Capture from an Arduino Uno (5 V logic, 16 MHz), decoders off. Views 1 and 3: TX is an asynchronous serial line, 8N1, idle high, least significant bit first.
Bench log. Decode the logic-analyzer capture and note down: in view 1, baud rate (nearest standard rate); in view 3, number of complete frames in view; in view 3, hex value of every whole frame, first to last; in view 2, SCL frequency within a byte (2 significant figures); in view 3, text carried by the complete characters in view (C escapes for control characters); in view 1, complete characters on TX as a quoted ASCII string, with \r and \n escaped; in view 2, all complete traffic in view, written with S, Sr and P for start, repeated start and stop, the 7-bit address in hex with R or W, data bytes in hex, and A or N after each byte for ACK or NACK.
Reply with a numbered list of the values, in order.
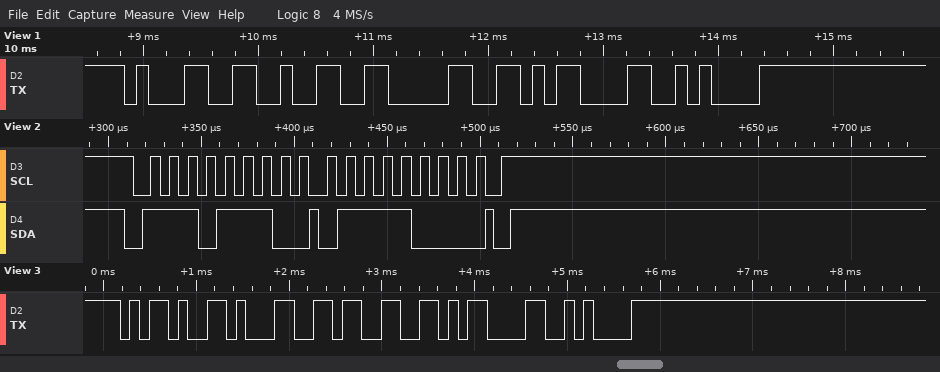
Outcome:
1. 9600 baud
2. 5
3. 0x2D 0x31 0x33 0x0D 0x0A
4. 100 kHz
5. "-13\r\n"
6. "120\r\n"
7. S 77W A 78 A P
